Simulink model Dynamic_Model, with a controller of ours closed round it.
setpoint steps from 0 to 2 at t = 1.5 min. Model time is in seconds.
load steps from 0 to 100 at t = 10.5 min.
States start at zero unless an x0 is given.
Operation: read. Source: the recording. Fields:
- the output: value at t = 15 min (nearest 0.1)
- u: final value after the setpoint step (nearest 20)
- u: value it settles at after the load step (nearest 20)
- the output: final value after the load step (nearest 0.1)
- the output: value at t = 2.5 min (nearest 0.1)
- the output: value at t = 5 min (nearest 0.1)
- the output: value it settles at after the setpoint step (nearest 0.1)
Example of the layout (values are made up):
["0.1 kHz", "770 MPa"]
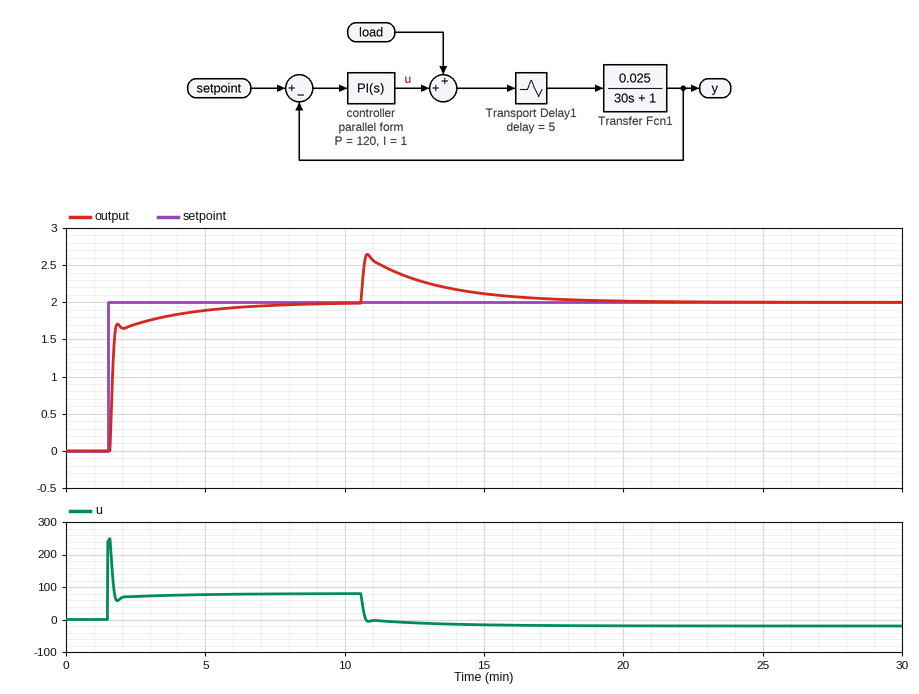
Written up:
["2.1", "80", "-20", "2.0", "1.7", "1.9", "2.0"]
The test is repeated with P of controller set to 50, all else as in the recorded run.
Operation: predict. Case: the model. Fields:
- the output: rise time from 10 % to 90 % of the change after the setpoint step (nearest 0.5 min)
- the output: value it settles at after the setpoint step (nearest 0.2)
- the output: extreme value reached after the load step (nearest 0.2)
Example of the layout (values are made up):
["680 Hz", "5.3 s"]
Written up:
["1.5 min", "2.0", "3.0"]
